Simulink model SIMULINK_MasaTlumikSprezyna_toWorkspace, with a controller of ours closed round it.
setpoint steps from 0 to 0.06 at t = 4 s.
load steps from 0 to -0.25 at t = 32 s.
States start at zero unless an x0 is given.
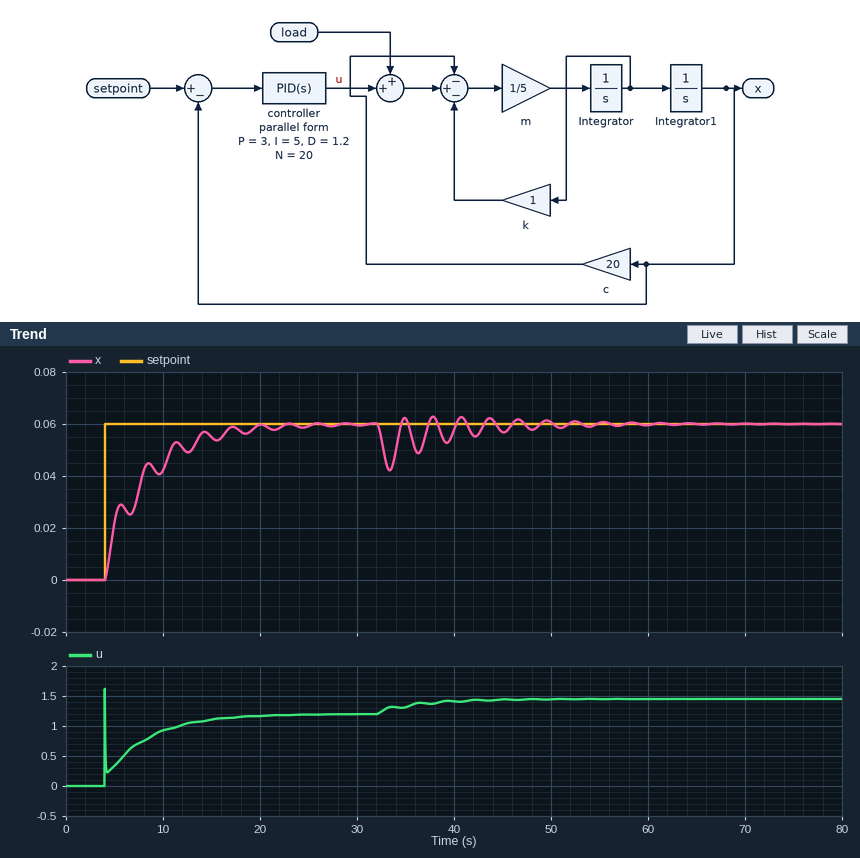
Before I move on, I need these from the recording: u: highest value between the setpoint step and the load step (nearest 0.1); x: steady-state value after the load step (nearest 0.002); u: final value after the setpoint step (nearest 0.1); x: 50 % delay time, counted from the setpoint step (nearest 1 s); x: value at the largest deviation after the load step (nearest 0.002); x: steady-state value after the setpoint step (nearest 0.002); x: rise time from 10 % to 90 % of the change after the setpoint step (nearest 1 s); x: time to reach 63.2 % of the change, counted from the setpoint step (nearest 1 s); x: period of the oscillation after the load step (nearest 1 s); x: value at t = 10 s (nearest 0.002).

1.6
0.060
1.2
3 s
0.042
0.060
9 s
4 s
3 s
0.042
